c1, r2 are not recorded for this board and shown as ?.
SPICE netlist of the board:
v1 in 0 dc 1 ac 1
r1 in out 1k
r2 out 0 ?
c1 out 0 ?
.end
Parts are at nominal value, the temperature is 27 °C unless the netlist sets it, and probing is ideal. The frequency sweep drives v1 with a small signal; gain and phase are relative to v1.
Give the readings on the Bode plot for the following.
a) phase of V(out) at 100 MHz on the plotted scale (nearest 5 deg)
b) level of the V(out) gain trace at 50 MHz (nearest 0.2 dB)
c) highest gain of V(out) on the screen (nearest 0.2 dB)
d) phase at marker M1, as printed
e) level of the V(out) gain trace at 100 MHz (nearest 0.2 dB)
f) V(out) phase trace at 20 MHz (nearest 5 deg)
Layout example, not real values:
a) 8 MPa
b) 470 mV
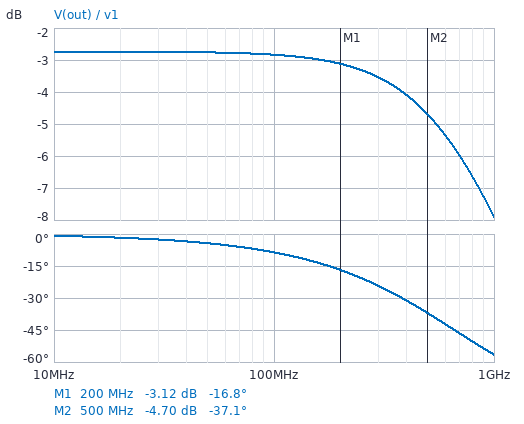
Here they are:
a) -10 deg
b) -2.8 dB
c) -2.8 dB
d) -16.8 deg
e) -2.8 dB
f) 0 deg
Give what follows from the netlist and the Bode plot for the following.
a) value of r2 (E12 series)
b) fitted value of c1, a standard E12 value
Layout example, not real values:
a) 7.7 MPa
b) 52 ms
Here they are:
a) 2.7 kΩ
b) 330 fF
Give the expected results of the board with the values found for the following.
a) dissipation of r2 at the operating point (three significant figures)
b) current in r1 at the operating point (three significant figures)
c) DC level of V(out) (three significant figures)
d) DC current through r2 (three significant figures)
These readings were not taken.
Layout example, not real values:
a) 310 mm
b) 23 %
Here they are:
a) 197 µW
b) 270 µA
c) 730 mV
d) 270 µA
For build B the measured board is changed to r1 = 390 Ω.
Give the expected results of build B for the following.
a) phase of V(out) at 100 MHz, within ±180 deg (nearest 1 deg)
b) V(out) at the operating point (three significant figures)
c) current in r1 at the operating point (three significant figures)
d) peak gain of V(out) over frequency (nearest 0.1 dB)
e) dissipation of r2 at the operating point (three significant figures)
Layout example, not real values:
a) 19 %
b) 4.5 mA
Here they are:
a) -4 deg
b) 874 mV
c) 324 µA
d) -1.2 dB
e) 283 µW
